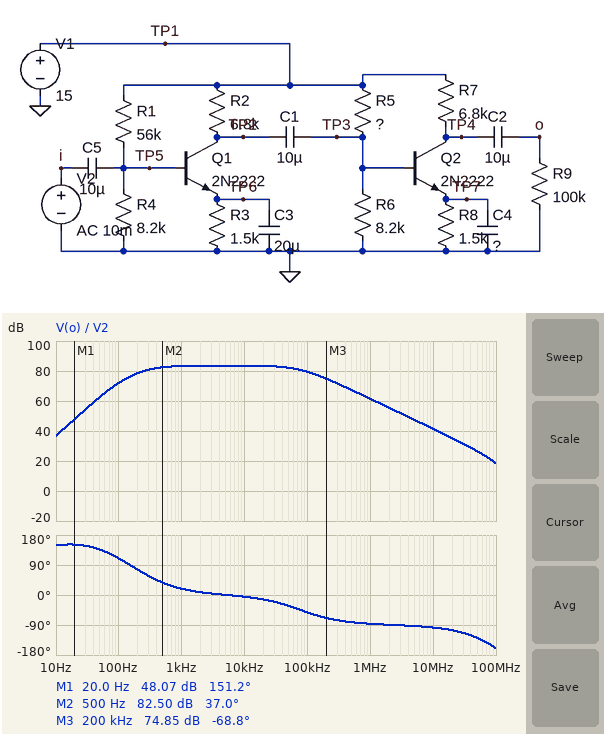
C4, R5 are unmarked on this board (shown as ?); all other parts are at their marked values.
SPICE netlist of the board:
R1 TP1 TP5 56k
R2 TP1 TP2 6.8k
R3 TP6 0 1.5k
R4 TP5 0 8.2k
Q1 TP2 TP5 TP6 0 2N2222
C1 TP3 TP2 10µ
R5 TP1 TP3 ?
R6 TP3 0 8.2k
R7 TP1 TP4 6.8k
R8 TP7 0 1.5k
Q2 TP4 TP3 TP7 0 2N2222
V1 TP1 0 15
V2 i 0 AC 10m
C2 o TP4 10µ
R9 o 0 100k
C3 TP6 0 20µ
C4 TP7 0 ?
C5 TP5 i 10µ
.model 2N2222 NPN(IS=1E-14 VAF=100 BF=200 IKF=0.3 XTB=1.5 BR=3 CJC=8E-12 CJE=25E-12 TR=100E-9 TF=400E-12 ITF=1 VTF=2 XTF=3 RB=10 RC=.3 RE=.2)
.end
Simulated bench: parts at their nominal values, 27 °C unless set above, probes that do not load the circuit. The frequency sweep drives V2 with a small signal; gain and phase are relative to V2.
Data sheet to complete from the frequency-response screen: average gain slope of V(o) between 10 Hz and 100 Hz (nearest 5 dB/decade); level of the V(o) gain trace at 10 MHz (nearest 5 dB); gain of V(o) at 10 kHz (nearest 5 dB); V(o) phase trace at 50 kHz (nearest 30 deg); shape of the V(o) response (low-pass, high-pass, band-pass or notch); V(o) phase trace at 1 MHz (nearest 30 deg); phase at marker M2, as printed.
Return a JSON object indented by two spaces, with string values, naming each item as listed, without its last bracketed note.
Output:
{
  "average gain slope of V(o) between 10 Hz and 100 Hz": "35 dB/decade",
  "level of the V(o) gain trace at 10 MHz": "40 dB",
  "gain of V(o) at 10 kHz": "85 dB",
  "V(o) phase trace at 50 kHz": "-30 deg",
  "shape of the V(o) response": "band-pass",
  "V(o) phase trace at 1 MHz": "-90 deg",
  "phase at marker M2, as printed": "37.0 deg"
}
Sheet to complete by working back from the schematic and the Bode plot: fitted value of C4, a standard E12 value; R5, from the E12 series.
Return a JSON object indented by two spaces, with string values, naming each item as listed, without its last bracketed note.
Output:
{
  "fitted value of C4, a standard E12 value": "39 µF",
  "R5, from the E12 series": "47 kΩ"
}
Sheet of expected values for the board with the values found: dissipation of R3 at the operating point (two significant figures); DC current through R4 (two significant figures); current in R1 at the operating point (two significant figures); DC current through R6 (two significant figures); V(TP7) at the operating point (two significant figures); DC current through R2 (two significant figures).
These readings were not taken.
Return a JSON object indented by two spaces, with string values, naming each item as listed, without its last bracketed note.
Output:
{
  "dissipation of R3 at the operating point": "1.0 mW",
  "DC current through R4": "230 µA",
  "current in R1 at the operating point": "230 µA",
  "DC current through R6": "270 µA",
  "V(TP7) at the operating point": "1.5 V",
  "DC current through R2": "820 µA"
}
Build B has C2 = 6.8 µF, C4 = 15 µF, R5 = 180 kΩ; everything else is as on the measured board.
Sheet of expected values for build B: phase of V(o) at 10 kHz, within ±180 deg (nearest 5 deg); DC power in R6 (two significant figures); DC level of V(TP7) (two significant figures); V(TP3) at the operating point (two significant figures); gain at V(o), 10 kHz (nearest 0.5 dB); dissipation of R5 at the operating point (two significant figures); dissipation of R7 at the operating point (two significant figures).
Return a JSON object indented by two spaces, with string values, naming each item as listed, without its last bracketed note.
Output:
{
  "phase of V(o) at 10 kHz, within ±180 deg": "0 deg",
  "DC power in R6": "52 µW",
  "DC level of V(TP7)": "77 mV",
  "V(TP3) at the operating point": "650 mV",
  "gain at V(o), 10 kHz": "62.5 dB",
  "dissipation of R5 at the operating point": "1.1 mW",
  "dissipation of R7 at the operating point": "18 µW"
}
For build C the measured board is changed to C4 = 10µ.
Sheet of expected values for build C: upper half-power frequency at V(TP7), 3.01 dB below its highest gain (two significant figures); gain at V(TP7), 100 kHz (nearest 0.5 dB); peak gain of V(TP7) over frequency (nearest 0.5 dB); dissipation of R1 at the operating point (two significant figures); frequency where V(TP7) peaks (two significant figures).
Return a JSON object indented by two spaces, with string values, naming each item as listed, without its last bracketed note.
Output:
{
  "upper half-power frequency at V(TP7), 3.01 dB below its highest gain": "760 Hz",
  "gain at V(TP7), 100 kHz": "-12.5 dB",
  "peak gain of V(TP7) over frequency": "35.5 dB",
  "dissipation of R1 at the operating point": "3.1 mW",
  "frequency where V(TP7) peaks": "310 Hz"
}
